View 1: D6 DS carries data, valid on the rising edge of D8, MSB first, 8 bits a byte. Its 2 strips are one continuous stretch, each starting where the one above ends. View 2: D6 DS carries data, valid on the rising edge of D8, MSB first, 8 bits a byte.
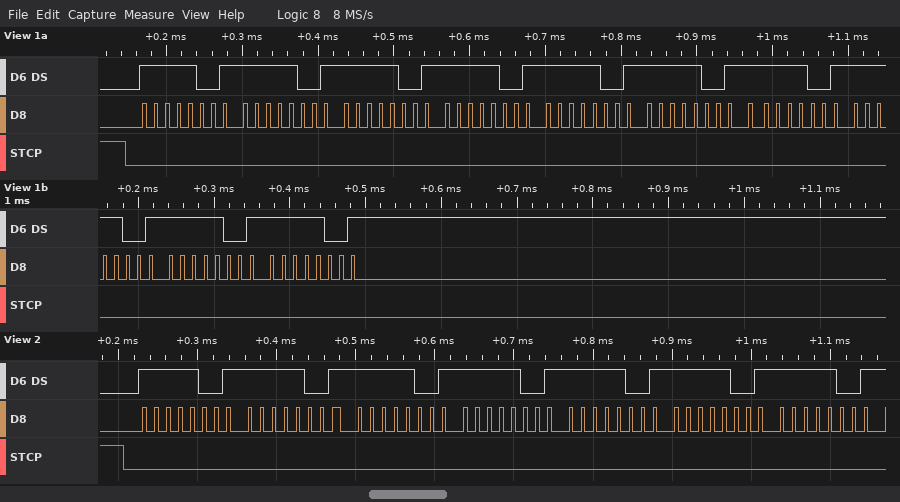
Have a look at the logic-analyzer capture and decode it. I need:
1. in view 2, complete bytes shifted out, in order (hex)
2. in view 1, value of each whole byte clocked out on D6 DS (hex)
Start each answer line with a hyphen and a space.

- F9 F9 F9 F9 F9 F9 F9
- F9 F9 F9 F9 F9 F9 F9 F9 F9 F9
